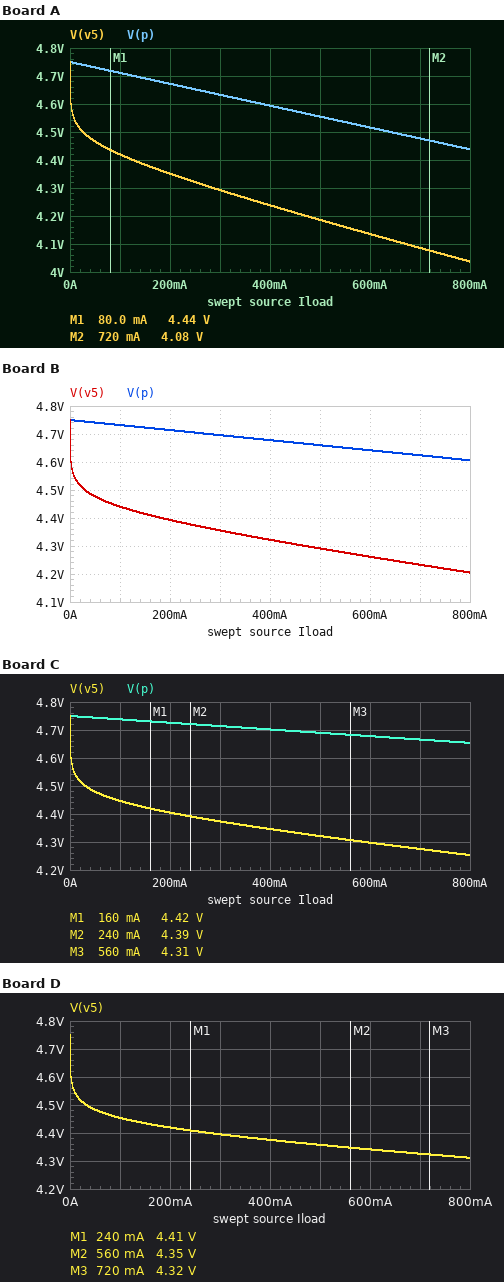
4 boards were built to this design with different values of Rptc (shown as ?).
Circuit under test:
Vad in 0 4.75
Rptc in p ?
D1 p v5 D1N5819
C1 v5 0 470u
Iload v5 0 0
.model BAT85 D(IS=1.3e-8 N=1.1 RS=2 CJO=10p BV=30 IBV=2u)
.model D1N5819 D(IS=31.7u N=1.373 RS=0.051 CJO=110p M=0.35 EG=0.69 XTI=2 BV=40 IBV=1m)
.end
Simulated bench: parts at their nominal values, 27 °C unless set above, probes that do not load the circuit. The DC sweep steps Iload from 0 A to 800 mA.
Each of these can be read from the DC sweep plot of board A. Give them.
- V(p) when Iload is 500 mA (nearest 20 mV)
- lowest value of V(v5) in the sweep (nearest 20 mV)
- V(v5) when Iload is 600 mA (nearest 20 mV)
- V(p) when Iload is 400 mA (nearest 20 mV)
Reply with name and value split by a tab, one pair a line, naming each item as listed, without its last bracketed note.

V(p) when Iload is 500 mA	4.56 V
lowest value of V(v5) in the sweep	4.04 V
V(v5) when Iload is 600 mA	4.14 V
V(p) when Iload is 400 mA	4.60 V
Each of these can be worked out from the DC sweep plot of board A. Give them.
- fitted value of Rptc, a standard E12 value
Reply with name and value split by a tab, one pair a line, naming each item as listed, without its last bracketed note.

fitted value of Rptc, a standard E12 value	0.39 Ω
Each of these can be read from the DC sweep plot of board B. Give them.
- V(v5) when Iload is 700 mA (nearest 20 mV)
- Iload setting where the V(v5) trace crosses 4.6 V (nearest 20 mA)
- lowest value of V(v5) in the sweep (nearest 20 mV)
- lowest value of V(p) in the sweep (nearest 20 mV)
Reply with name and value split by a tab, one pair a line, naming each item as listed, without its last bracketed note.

V(v5) when Iload is 700 mA	4.24 V
Iload setting where the V(v5) trace crosses 4.6 V	0 A
lowest value of V(v5) in the sweep	4.20 V
lowest value of V(p) in the sweep	4.60 V
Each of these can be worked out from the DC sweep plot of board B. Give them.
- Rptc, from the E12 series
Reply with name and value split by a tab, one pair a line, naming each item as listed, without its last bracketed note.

Rptc, from the E12 series	0.18 Ω
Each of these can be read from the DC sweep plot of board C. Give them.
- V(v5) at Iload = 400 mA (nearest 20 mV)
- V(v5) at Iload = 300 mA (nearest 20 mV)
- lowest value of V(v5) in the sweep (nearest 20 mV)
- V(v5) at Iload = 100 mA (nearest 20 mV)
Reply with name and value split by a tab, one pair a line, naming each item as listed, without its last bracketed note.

V(v5) at Iload = 400 mA	4.34 V
V(v5) at Iload = 300 mA	4.38 V
lowest value of V(v5) in the sweep	4.26 V
V(v5) at Iload = 100 mA	4.44 V
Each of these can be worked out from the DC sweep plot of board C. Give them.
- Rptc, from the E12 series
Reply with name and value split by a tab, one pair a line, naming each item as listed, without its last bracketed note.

Rptc, from the E12 series	0.12 Ω
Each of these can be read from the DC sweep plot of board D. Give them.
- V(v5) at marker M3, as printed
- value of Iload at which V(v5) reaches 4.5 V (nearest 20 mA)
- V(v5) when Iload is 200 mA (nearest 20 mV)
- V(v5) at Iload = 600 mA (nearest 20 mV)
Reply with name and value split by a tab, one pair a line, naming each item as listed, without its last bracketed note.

V(v5) at marker M3, as printed	4.32 V
value of Iload at which V(v5) reaches 4.5 V	40 mA
V(v5) when Iload is 200 mA	4.42 V
V(v5) at Iload = 600 mA	4.34 V
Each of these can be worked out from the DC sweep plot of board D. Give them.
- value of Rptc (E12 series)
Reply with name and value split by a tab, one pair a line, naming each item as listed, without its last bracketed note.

value of Rptc	0.047 Ω
